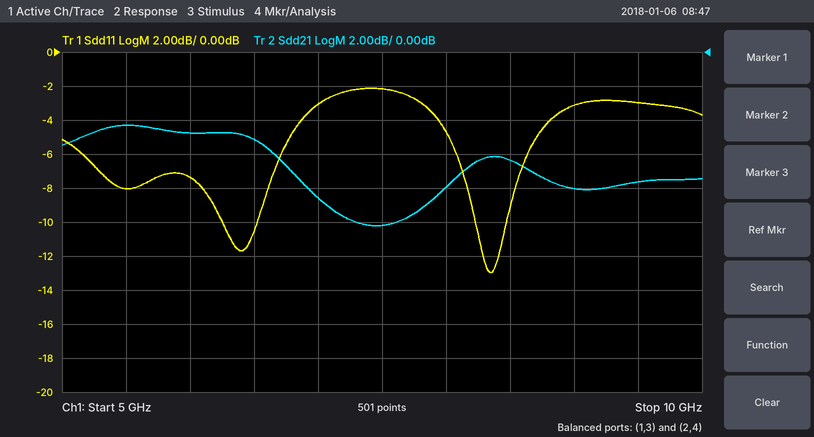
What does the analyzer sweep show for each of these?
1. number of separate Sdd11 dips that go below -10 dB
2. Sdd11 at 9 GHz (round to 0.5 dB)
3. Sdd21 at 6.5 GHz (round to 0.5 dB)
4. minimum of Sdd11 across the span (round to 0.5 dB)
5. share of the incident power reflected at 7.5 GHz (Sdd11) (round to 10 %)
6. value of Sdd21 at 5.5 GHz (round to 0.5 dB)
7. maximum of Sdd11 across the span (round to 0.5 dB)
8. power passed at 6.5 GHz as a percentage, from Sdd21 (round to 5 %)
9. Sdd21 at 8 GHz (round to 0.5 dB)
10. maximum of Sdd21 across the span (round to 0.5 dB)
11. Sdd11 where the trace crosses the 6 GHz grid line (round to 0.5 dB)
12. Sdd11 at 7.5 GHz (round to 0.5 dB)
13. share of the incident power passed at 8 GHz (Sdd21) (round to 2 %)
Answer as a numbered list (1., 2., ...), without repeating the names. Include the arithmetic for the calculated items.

1. 2
2. -3.0 dB
3. -5.0 dB
4. -13.0 dB
5. 10^(-2/10) ≈ 63.1 %, so 60 % to the nearest 10 %
6. -4.5 dB
7. -2.0 dB
8. 10^(-5/10) ≈ 31.6 %, so 30 % to the nearest 5 %
9. -8.0 dB
10. -4.5 dB
11. -7.5 dB
12. -2.0 dB
13. 10^(-8/10) ≈ 16 %
